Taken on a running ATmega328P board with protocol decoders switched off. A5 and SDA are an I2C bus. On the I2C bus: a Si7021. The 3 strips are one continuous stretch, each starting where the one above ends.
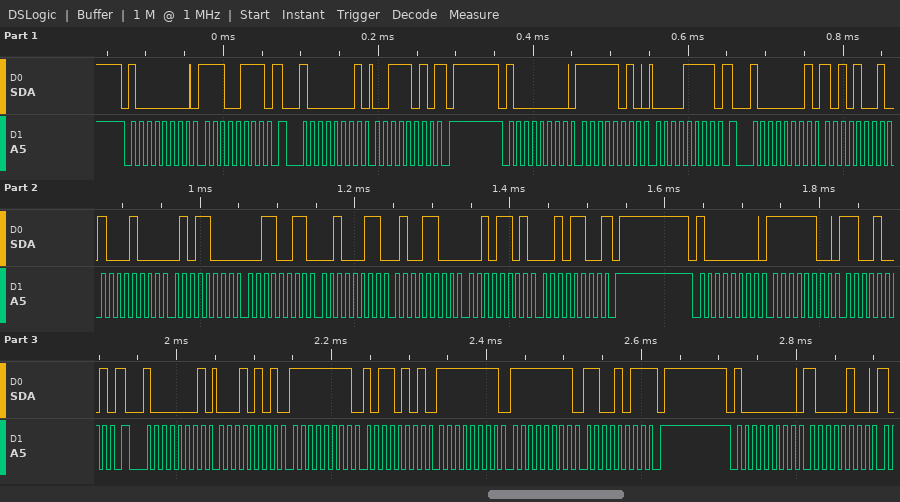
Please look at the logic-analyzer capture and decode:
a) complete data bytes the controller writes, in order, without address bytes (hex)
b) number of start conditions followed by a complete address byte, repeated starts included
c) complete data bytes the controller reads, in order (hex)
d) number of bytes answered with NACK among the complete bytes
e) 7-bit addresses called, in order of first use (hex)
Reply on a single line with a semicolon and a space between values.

E7 FA 0F FC C9 84; 7; 3A A9 88 58 33 23 4C 2D 2C 15 FF B5 FF FF CB; 3; 0x40
